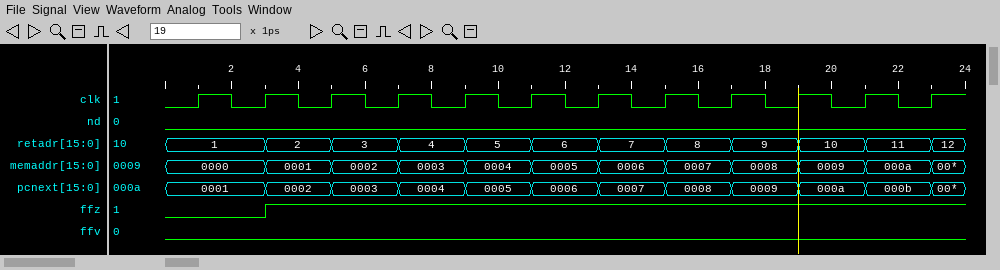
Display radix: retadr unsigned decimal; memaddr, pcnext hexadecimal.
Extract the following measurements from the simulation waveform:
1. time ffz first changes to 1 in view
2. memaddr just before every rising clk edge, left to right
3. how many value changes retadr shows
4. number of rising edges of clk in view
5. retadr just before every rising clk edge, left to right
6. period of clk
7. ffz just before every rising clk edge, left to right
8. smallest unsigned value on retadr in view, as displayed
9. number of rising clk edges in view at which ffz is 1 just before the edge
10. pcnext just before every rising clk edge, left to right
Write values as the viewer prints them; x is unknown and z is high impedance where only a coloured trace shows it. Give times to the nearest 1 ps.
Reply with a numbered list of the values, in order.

1. 3 ps
2. 0000, 0000, 0001, 0002, 0003, 0004, 0005, 0006, 0007, 0008, 0009, 000a
3. 11
4. 12
5. 1, 1, 2, 3, 4, 5, 6, 7, 8, 9, 10, 11
6. 2 ps
7. 0 0 1 1 1 1 1 1 1 1 1 1
8. 1
9. 10
10. 0001, 0001, 0002, 0003, 0004, 0005, 0006, 0007, 0008, 0009, 000a, 000b
